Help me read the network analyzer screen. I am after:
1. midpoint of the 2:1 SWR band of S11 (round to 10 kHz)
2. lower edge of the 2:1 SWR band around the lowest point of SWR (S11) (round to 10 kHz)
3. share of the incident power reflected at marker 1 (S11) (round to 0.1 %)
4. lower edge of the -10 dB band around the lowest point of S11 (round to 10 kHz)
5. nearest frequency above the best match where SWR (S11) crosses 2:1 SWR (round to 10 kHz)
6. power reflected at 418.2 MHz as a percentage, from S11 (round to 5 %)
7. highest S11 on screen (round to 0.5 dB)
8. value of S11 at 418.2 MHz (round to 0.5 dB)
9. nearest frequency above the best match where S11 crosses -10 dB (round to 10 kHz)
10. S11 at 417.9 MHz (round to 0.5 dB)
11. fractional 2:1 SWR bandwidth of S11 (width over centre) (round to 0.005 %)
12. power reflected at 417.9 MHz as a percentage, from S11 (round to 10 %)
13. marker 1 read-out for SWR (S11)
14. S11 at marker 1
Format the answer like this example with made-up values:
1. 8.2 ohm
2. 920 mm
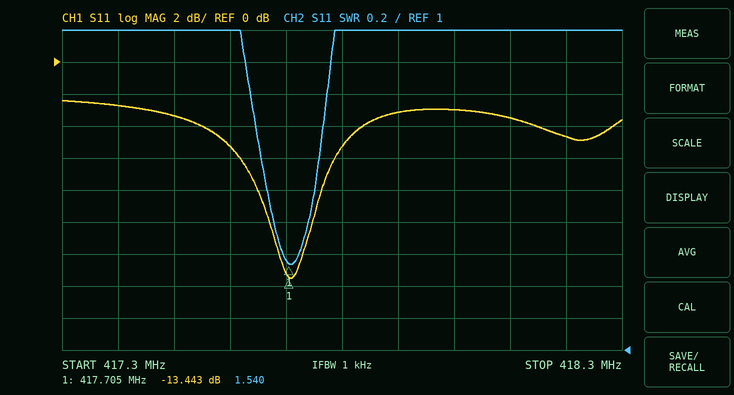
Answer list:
1. 417.71 MHz
2. 417.67 MHz
3. 4.5 %
4. 417.67 MHz
5. 417.75 MHz
6. 35 %
7. -2.5 dB
8. -4.5 dB
9. 417.75 MHz
10. -3.0 dB
11. 0.020 %
12. 50 %
13. 1.540
14. -13.443 dB
